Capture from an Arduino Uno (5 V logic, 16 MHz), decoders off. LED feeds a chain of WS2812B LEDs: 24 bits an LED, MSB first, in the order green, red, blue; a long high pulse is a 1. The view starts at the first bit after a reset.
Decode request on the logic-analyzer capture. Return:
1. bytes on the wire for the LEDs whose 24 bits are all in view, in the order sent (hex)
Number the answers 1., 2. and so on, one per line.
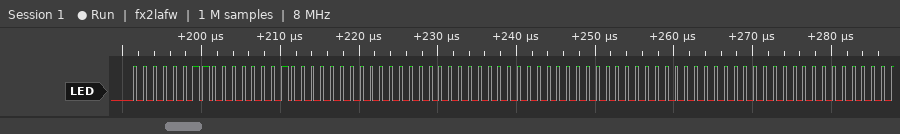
1. 03 01 00 00 00 00 00 00 00
